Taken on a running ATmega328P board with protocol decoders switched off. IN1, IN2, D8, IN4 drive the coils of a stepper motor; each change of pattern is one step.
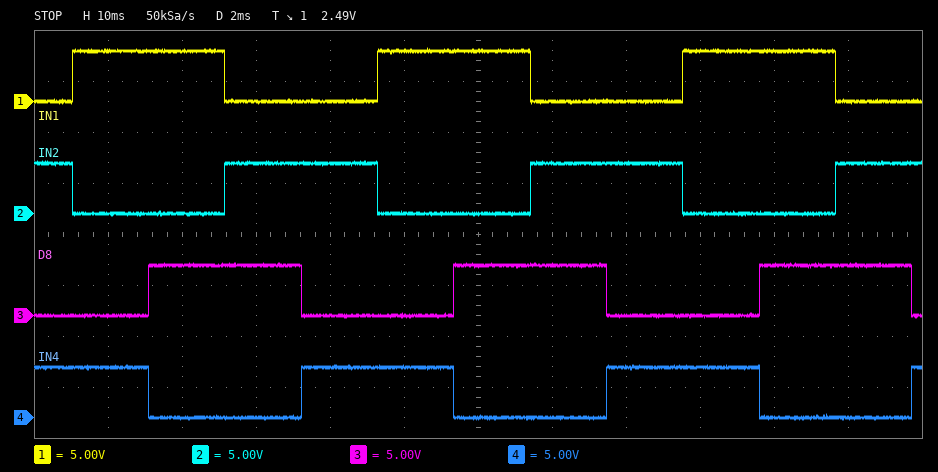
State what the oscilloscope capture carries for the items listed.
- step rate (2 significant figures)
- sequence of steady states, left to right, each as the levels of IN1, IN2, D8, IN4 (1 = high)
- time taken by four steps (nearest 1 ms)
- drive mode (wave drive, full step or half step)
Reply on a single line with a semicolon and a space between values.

97 steps/s; 0101 1001 1010 0110 0101 1001 1010 0110 0101 1001 1010 0110 0101; 41 ms; full step
